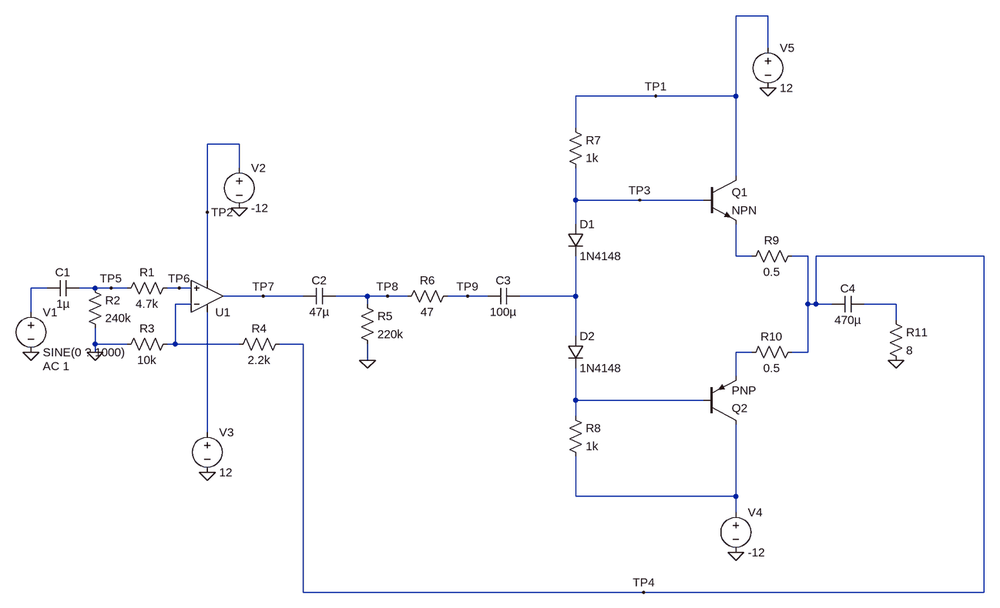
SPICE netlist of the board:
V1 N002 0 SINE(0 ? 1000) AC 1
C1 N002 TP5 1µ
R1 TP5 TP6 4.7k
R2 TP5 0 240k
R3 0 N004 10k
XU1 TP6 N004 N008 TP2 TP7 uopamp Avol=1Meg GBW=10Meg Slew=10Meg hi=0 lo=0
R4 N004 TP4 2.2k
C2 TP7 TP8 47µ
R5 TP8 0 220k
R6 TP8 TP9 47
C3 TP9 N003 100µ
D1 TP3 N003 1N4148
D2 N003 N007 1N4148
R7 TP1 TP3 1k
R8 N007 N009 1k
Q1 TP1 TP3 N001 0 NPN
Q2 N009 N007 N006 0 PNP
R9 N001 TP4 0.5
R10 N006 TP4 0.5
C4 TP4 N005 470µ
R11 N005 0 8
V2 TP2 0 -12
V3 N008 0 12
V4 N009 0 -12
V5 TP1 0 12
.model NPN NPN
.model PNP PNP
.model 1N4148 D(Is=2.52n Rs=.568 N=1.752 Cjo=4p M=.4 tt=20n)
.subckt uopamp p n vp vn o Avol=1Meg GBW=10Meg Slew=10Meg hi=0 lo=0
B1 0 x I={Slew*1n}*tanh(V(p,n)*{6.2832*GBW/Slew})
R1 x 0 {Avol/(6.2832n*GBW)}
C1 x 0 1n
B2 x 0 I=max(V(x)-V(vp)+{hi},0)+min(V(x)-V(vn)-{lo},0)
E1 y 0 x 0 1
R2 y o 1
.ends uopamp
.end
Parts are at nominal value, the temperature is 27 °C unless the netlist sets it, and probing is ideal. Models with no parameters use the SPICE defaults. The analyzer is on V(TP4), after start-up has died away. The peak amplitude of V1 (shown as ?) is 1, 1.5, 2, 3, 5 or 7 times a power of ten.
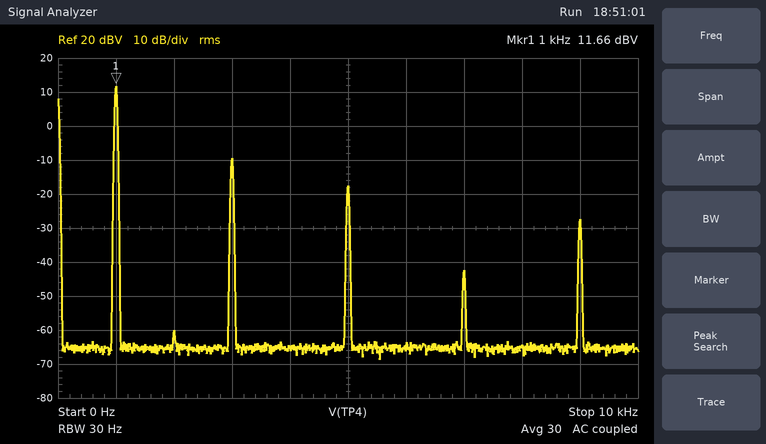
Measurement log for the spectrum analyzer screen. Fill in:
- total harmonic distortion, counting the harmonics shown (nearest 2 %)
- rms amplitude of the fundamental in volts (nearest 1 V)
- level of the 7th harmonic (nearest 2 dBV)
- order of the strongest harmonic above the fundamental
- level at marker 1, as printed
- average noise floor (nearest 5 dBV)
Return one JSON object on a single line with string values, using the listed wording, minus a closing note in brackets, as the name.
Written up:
{"total harmonic distortion, counting the harmonics shown": "10 %", "rms amplitude of the fundamental in volts": "4 V", "level of the 7th harmonic": "-42 dBV", "order of the strongest harmonic above the fundamental": "3", "level at marker 1, as printed": "11.66 dBV", "average noise floor": "-65 dBV"}
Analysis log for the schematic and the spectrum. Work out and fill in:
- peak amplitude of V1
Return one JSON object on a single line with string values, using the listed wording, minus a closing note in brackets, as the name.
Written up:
{"peak amplitude of V1": "5 V"}
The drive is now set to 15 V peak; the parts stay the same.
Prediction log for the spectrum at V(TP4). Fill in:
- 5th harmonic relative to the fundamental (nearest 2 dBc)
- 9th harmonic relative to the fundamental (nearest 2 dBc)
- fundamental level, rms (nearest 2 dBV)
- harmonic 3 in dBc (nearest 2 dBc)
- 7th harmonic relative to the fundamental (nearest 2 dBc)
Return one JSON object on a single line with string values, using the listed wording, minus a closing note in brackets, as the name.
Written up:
{"5th harmonic relative to the fundamental": "-16 dBc", "9th harmonic relative to the fundamental": "-30 dBc", "fundamental level, rms": "12 dBV", "harmonic 3 in dBc": "-10 dBc", "7th harmonic relative to the fundamental": "-22 dBc"}
